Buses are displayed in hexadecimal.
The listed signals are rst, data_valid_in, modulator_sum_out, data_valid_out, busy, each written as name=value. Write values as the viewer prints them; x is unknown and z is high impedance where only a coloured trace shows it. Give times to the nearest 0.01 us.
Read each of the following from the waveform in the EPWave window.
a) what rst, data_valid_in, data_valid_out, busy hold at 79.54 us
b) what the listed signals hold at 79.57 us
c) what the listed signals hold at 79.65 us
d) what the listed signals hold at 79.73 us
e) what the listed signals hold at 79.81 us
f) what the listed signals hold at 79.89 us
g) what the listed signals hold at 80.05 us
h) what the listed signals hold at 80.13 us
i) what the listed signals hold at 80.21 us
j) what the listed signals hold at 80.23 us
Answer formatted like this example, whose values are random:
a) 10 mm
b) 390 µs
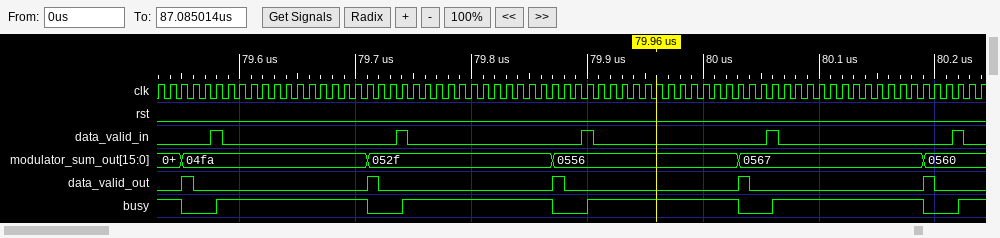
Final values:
a) rst=0, data_valid_in=0, data_valid_out=0, busy=1
b) rst=0, data_valid_in=0, modulator_sum_out=04fa, data_valid_out=0, busy=0
c) rst=0, data_valid_in=0, modulator_sum_out=04fa, data_valid_out=0, busy=1
d) rst=0, data_valid_in=0, modulator_sum_out=052f, data_valid_out=0, busy=0
e) rst=0, data_valid_in=0, modulator_sum_out=052f, data_valid_out=0, busy=1
f) rst=0, data_valid_in=0, modulator_sum_out=0556, data_valid_out=0, busy=0
g) rst=0, data_valid_in=0, modulator_sum_out=0567, data_valid_out=0, busy=0
h) rst=0, data_valid_in=0, modulator_sum_out=0567, data_valid_out=0, busy=1
i) rst=0, data_valid_in=0, modulator_sum_out=0560, data_valid_out=0, busy=0
j) rst=0, data_valid_in=0, modulator_sum_out=0560, data_valid_out=0, busy=1
